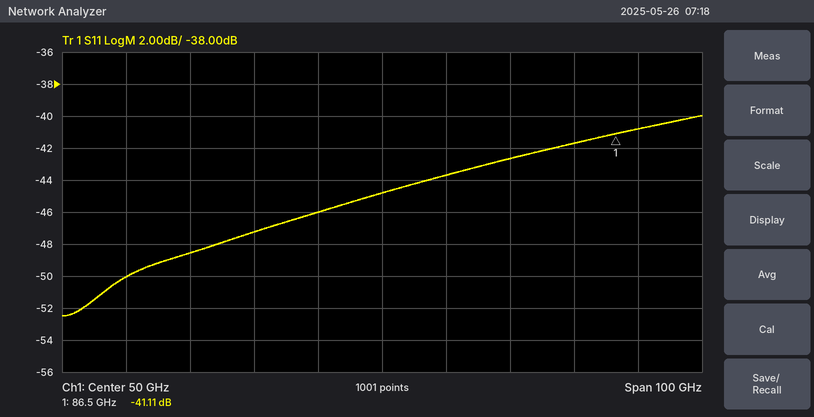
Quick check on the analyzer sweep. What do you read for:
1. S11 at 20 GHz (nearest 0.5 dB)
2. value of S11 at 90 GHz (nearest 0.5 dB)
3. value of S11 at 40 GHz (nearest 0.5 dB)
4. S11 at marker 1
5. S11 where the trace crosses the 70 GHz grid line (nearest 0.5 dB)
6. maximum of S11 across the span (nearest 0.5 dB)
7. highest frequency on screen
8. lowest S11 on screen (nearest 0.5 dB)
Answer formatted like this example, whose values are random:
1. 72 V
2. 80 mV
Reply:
1. -48.5 dB
2. -41.0 dB
3. -46.0 dB
4. -41.11 dB
5. -42.5 dB
6. -40.0 dB
7. 100 GHz
8. -52.5 dB
